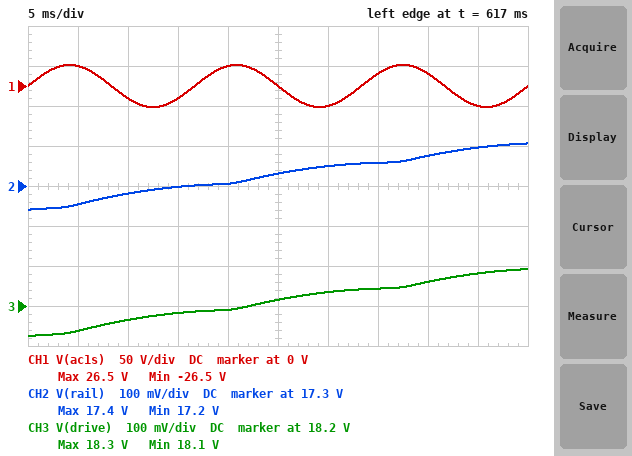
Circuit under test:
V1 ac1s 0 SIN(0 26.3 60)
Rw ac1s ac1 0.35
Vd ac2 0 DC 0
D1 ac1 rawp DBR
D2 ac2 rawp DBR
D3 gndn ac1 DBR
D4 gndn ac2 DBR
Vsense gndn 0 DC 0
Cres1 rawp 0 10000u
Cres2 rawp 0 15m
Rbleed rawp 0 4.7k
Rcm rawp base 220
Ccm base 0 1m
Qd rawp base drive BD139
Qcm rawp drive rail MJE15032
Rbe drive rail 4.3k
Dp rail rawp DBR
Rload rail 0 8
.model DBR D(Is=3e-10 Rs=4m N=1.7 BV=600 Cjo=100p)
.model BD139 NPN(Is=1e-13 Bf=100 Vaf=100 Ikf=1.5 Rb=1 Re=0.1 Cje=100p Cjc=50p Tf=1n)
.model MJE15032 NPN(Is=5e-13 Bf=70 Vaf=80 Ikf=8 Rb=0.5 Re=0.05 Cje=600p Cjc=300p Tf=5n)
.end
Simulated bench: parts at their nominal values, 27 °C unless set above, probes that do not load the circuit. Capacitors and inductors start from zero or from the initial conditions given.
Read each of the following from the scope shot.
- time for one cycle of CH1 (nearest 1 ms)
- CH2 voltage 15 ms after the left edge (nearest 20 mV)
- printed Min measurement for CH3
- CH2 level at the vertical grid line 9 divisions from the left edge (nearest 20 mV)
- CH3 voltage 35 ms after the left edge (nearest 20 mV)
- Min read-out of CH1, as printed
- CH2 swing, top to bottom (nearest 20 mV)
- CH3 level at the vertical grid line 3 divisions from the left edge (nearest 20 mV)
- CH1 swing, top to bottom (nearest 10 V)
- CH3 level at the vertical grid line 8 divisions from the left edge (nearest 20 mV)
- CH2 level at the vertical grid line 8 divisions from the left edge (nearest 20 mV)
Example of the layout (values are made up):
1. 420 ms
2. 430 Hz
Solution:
1. 17 ms
2. 17.30 V
3. 18.1 V
4. 17.40 V
5. 18.24 V
6. -26.5 V
7. 160 mV
8. 18.18 V
9. 50 V
10. 18.26 V
11. 17.38 V
